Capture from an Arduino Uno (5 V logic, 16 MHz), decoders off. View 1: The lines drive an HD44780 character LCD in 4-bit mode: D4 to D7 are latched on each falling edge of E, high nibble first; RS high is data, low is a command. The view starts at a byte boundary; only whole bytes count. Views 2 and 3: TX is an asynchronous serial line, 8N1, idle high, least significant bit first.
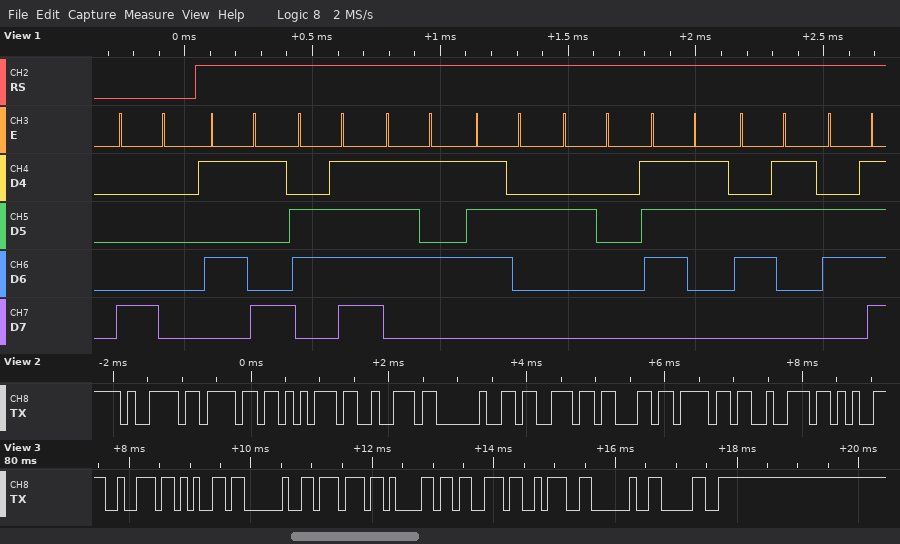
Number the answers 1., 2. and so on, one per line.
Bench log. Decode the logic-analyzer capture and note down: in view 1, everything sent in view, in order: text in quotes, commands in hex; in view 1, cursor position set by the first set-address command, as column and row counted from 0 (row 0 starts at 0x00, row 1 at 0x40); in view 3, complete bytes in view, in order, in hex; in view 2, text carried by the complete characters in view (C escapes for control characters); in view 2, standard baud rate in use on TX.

1. 0x80 "Your sco"
2. column 0, row 0
3. 72 65 20 77 61 73 3A 20 30
4. "your scor"
5. 9600 baud
